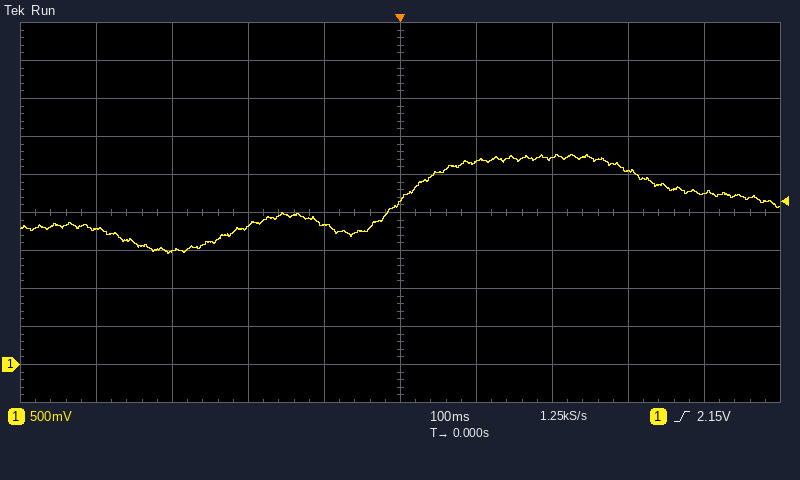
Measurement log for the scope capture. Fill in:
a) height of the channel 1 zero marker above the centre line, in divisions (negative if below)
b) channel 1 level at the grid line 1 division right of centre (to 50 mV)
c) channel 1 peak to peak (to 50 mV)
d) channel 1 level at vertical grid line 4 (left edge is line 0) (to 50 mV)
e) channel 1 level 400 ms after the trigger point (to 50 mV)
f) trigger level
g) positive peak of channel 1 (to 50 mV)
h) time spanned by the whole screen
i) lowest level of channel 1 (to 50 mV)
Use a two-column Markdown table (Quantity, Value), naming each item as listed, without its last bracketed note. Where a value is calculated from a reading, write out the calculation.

| Quantity | Value |
|---|---|
| height of the channel 1 zero marker above the centre line, in divisions | -4.0 div |
| channel 1 level at the grid line 1 division right of centre | 2.65 V |
| channel 1 peak to peak | 2.75 V − (1.45 V) = 1.30 V |
| channel 1 level at vertical grid line 4 (left edge is line 0) | 1.85 V |
| channel 1 level 400 ms after the trigger point | 2.25 V |
| trigger level | 2.15 V |
| positive peak of channel 1 | 2.75 V |
| time spanned by the whole screen | 1 s |
| lowest level of channel 1 | 1.45 V |
